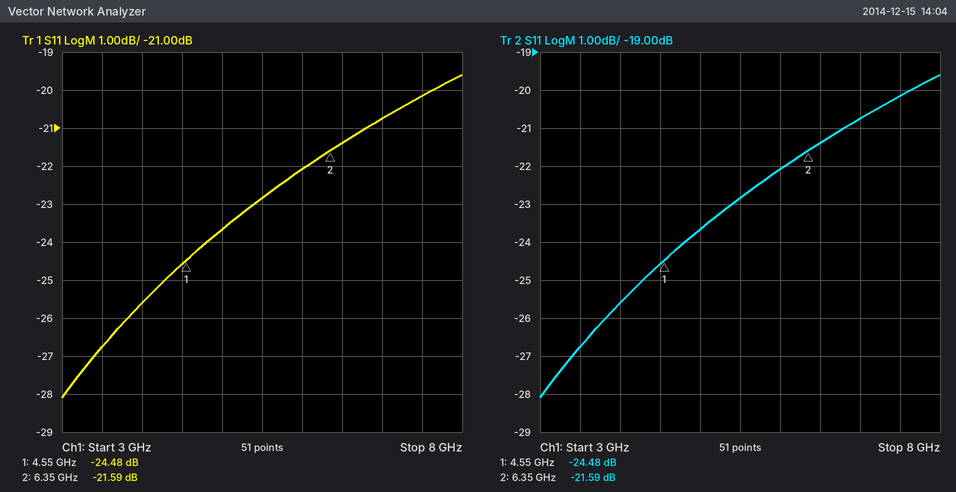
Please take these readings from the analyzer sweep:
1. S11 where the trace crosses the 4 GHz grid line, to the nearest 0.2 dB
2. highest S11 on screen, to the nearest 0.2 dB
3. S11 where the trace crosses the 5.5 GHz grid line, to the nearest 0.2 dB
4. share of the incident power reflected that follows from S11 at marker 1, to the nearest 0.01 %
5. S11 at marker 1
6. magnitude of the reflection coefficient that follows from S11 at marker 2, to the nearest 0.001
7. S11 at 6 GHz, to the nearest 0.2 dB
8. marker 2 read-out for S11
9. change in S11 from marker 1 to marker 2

-25.6 dB
-19.6 dB
-22.8 dB
0.36 %
-24.48 dB
0.083
-22.0 dB
-21.59 dB
2.89 dB
